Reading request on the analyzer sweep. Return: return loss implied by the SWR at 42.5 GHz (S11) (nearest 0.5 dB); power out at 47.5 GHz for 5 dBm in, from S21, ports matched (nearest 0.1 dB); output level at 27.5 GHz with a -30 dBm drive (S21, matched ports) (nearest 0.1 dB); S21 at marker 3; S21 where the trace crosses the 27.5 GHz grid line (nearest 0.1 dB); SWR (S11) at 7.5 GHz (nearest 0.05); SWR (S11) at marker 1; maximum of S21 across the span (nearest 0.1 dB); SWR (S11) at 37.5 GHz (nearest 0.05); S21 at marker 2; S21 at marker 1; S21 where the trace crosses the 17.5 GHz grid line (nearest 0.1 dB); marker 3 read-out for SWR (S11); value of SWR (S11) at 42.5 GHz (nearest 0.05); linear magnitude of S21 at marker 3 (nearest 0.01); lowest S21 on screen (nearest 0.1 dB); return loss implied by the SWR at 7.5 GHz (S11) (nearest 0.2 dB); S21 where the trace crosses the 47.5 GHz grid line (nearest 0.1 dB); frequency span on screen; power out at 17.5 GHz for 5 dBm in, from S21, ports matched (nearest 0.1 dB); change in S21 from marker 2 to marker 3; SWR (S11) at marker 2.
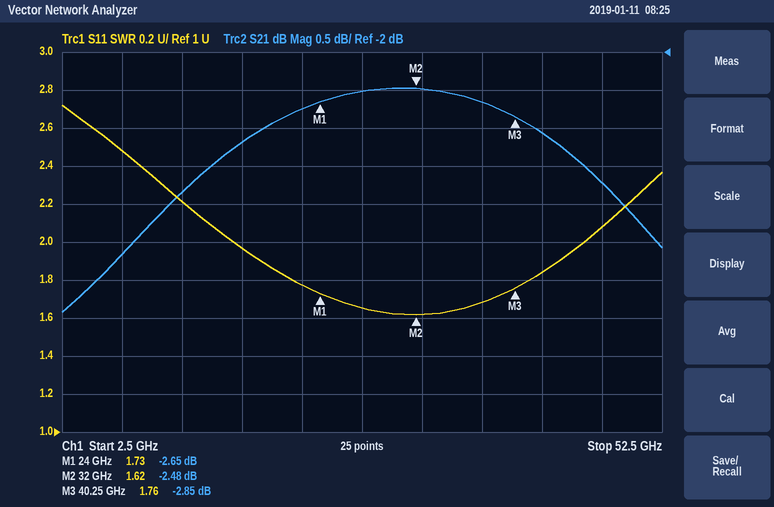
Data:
10.5 dB
1.3 dBm
-32.5 dBm
-2.85 dB
-2.5 dB
2.50
1.73
-2.5 dB
1.70
-2.48 dB
-2.65 dB
-3.2 dB
1.76
1.85
0.72
-5.4 dB
7.4 dB
-3.7 dB
50 GHz
1.8 dBm
-0.37 dB
1.62
